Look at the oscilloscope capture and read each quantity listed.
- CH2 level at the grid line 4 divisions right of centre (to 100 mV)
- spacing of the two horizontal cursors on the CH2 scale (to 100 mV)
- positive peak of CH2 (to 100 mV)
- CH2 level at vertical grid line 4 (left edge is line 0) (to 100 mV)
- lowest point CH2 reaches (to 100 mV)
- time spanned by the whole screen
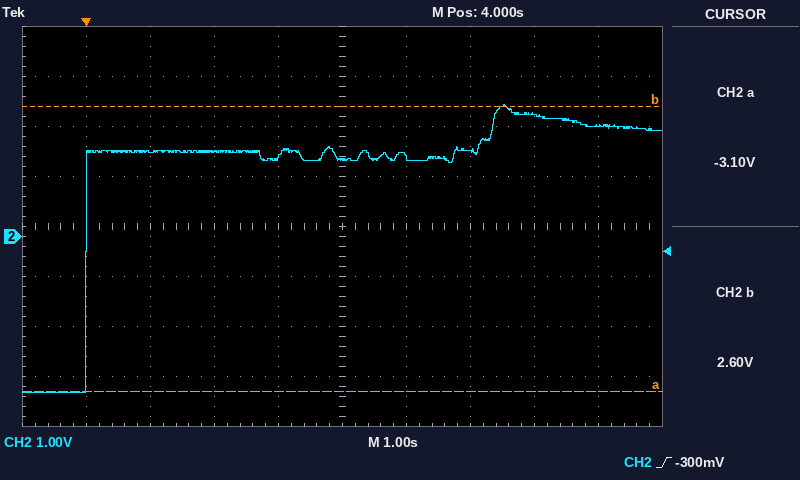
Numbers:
2.2 V
5.7 V
2.6 V
1.6 V
-3.1 V
10 s
